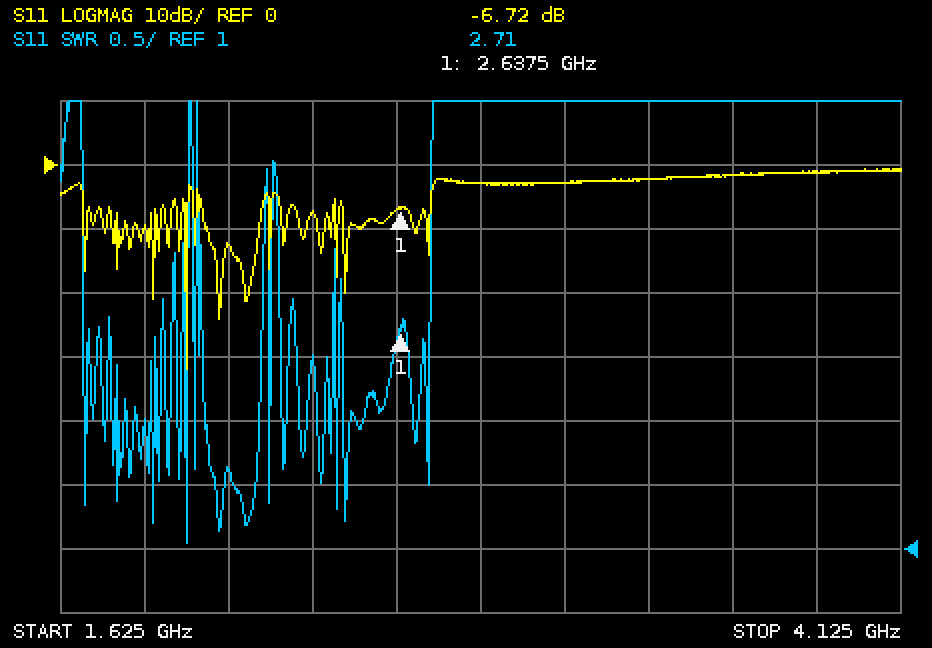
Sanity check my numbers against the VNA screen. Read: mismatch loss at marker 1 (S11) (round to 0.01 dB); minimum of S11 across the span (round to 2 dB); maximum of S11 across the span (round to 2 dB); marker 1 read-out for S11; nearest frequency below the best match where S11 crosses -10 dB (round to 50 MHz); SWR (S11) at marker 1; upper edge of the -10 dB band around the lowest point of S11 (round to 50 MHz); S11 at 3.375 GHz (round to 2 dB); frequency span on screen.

1.04 dB
-32 dB
0 dB
-6.72 dB
2.00 GHz
2.71
2.00 GHz
-2 dB
2.5 GHz
